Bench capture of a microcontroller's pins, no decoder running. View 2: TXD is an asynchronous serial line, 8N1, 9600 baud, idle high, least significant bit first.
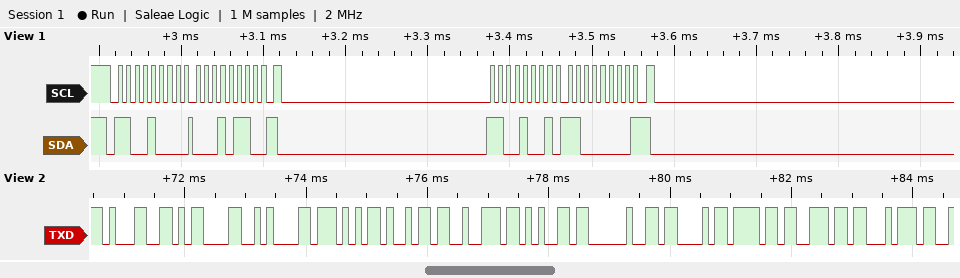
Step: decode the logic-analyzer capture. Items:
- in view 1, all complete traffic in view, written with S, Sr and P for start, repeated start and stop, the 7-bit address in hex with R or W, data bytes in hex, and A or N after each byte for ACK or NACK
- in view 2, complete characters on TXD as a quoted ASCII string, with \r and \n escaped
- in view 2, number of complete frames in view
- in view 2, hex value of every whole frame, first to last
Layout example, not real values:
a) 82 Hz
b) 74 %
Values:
a) S 64W A 16 A Sr 64R A C0 N
b) "1\r\nWire Cont"
c) 12
d) 0x31 0x0D 0x0A 0x57 0x69 0x72 0x65 0x20 0x43 0x6F 0x6E 0x74
